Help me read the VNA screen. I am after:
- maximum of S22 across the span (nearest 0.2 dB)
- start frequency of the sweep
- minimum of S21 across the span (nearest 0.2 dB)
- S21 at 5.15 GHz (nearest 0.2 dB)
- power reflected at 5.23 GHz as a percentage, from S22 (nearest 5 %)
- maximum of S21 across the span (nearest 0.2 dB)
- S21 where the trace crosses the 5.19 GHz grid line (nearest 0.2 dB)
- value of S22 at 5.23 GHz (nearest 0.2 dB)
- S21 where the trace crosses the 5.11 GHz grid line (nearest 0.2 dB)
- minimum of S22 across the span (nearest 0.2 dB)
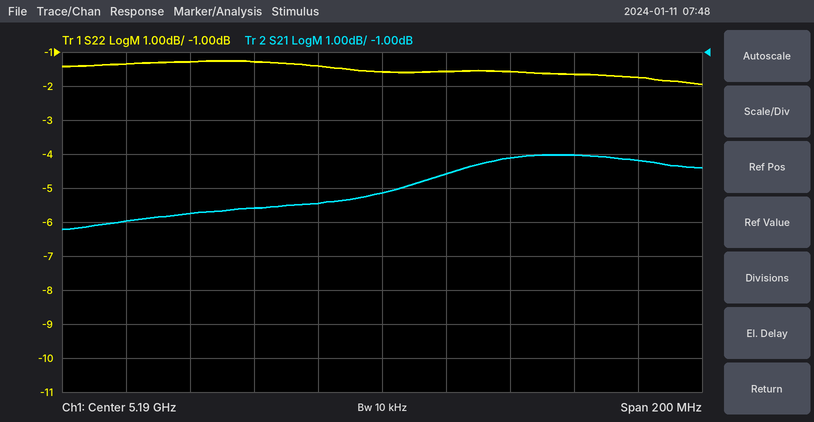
-1.2 dB
5.09 GHz
-6.2 dB
-5.6 dB
70 %
-4.0 dB
-5.2 dB
-1.6 dB
-6.0 dB
-2.0 dB
